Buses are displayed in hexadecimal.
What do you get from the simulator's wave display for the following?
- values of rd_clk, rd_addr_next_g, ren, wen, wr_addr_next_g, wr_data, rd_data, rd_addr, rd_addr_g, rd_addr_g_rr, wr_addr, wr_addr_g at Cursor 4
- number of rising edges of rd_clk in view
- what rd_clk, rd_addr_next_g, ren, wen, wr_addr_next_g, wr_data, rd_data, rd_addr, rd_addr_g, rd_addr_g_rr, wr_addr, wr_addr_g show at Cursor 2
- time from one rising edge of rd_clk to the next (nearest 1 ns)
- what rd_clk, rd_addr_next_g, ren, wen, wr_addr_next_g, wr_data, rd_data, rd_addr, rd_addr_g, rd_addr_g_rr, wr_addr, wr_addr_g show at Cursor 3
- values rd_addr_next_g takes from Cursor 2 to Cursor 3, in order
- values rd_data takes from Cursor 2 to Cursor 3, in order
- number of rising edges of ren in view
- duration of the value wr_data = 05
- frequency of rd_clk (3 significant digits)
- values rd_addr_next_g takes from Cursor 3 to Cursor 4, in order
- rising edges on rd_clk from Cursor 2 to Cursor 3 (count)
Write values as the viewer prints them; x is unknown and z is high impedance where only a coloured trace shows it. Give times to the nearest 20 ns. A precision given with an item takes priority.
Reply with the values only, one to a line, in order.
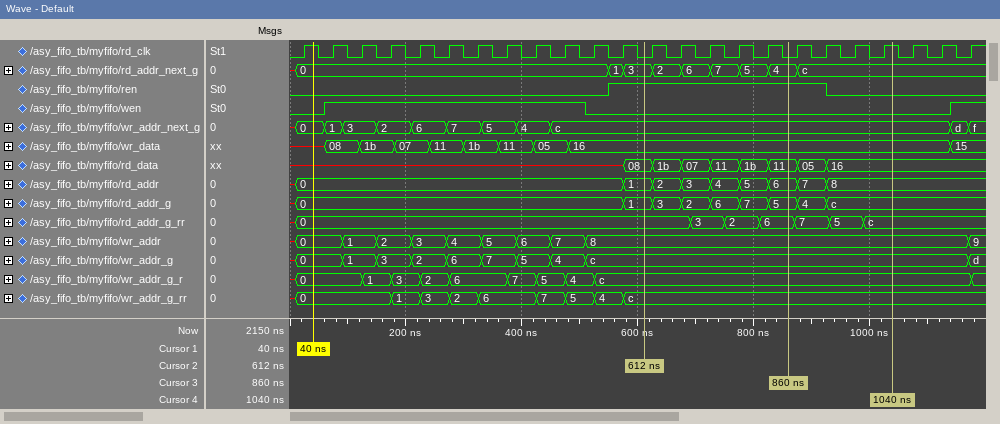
rd_clk=1, rd_addr_next_g=c, ren=0, wen=0, wr_addr_next_g=c, wr_data=16, rd_data=16, rd_addr=8, rd_addr_g=c, rd_addr_g_rr=c, wr_addr=8, wr_addr_g=c
24
rd_clk=0, rd_addr_next_g=3, ren=1, wen=0, wr_addr_next_g=c, wr_data=16, rd_data=08, rd_addr=1, rd_addr_g=1, rd_addr_g_rr=0, wr_addr=8, wr_addr_g=c
50 ns
rd_clk=0, rd_addr_next_g=4, ren=1, wen=0, wr_addr_next_g=c, wr_data=16, rd_data=11, rd_addr=6, rd_addr_g=5, rd_addr_g_rr=6, wr_addr=8, wr_addr_g=c
3, 2, 6, 7, 5, 4
08, 1b, 07, 11, 1b, 11
1
60 ns
20.0 MHz
4, c
5
